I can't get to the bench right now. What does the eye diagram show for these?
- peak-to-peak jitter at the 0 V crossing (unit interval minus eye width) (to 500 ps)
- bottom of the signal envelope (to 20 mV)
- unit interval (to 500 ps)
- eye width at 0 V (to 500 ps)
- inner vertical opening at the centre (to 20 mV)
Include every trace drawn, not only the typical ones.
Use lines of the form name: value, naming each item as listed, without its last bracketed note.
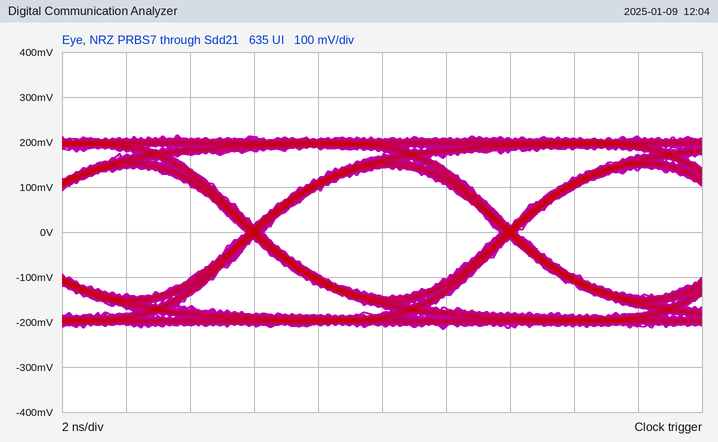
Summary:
peak-to-peak jitter at the 0 V crossing (unit interval minus eye width): 500 ps
bottom of the signal envelope: -220 mV
unit interval: 8.0 ns
eye width at 0 V: 7.5 ns
inner vertical opening at the centre: 280 mV
